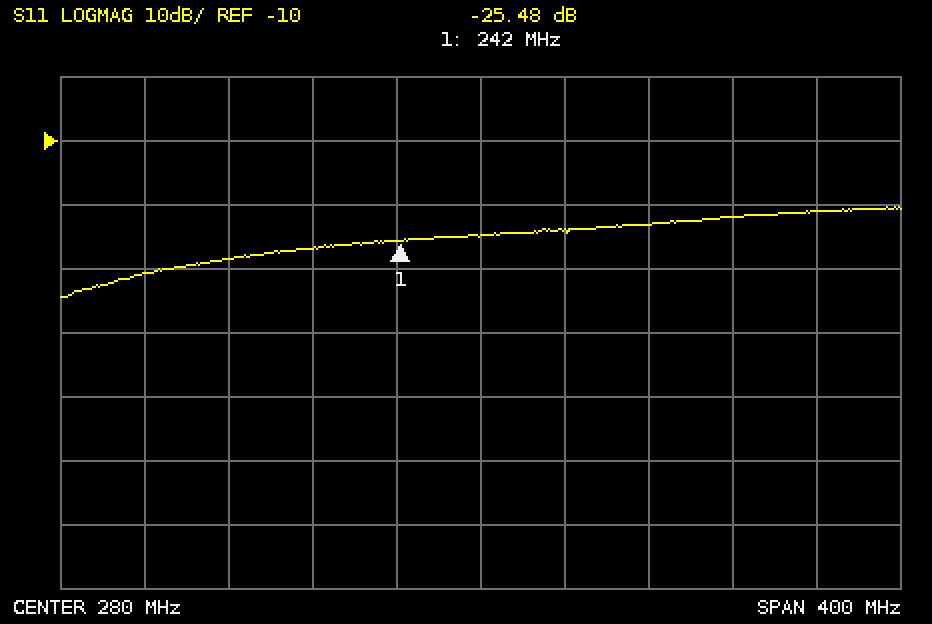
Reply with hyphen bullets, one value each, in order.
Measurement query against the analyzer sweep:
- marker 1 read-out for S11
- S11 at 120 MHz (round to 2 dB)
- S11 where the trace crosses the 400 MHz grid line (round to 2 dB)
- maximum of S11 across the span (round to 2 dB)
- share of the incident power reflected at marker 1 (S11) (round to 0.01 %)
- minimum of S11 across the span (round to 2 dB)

- -25.48 dB
- -30 dB
- -22 dB
- -20 dB
- 0.28 %
- -34 dB
